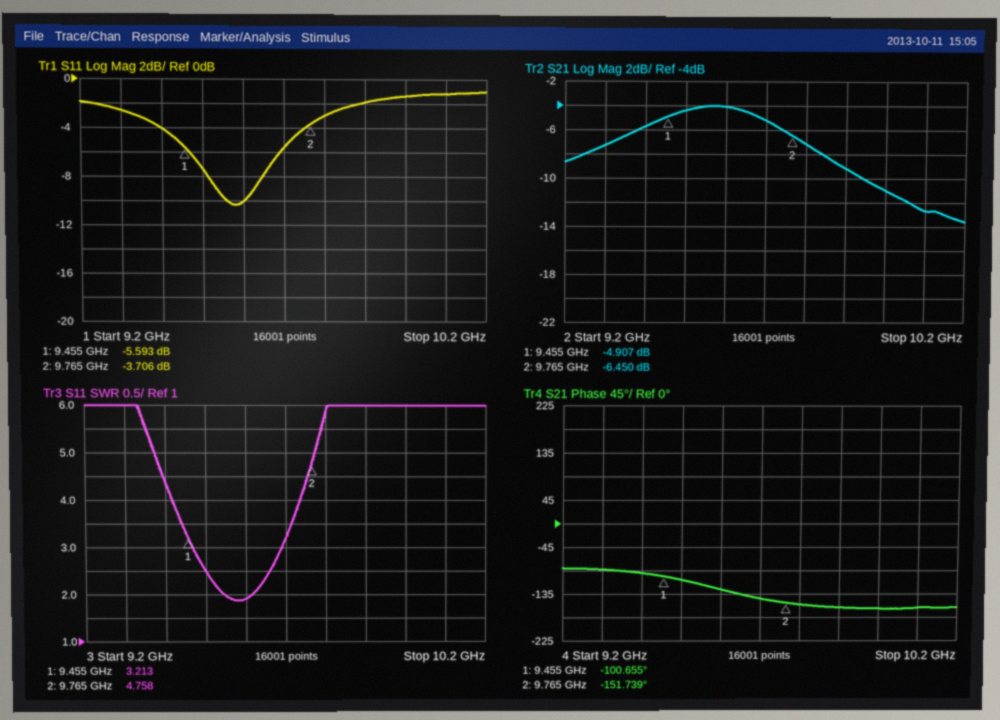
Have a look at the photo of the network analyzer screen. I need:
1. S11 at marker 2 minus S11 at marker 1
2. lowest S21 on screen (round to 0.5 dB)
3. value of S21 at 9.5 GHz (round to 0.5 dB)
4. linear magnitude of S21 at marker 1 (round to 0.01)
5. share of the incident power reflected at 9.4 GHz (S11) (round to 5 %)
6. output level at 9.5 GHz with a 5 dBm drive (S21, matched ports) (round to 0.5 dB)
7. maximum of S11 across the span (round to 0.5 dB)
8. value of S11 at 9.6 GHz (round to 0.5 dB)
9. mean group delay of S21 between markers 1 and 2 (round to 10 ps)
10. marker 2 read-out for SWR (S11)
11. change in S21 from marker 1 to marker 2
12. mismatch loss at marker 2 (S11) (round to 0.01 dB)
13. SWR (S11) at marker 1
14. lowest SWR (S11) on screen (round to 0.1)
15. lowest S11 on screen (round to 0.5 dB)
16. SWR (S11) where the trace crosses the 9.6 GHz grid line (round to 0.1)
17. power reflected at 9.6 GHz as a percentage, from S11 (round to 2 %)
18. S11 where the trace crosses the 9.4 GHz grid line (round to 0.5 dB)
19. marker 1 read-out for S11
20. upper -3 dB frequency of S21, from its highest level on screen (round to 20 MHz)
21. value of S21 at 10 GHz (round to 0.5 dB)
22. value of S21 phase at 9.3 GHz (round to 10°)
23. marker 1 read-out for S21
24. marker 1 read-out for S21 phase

1.887 dB
-13.5 dB
-4.5 dB
0.57
40 %
0.5 dBm
-1.0 dB
-10.0 dB
460 ps
4.758
-1.543 dB
2.41 dB
3.213
1.9
-10.5 dB
1.9
10 %
-4.0 dB
-5.593 dB
9.80 GHz
-11.0 dB
-90°
-4.907 dB
-100.655°
